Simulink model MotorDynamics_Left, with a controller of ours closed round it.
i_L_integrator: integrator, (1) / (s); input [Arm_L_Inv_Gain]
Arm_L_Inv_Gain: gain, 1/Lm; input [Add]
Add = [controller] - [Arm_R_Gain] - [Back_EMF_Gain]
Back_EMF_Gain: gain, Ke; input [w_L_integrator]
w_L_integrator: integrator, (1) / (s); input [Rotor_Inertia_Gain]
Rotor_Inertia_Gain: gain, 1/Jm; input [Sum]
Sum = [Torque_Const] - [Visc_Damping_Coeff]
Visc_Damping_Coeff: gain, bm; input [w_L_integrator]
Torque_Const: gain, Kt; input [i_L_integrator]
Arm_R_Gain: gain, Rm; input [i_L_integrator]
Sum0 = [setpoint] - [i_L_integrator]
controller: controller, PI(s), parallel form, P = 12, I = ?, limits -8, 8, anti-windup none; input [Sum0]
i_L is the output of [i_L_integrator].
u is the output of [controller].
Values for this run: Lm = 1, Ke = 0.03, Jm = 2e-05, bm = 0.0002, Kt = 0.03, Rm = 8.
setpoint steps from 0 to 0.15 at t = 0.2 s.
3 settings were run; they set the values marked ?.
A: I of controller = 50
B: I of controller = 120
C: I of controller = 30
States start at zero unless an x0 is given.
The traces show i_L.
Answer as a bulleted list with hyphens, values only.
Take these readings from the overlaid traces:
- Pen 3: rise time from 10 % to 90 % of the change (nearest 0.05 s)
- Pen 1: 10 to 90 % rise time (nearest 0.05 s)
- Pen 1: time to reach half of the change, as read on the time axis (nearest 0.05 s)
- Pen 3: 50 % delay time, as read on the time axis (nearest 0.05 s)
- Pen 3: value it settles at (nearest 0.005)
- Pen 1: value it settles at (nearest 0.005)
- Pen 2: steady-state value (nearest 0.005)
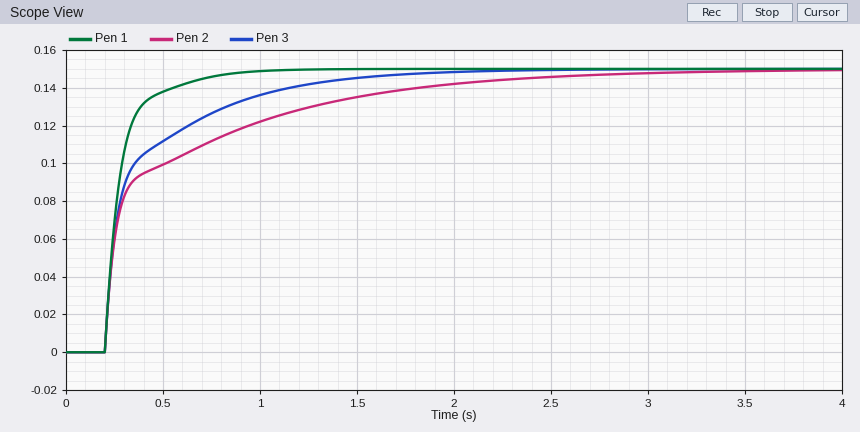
- 0.75 s
- 0.25 s
- 0.25 s
- 0.25 s
- 0.150
- 0.150
- 0.150
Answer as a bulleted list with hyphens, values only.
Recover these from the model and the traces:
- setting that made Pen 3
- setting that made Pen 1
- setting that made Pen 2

- A
- B
- C
